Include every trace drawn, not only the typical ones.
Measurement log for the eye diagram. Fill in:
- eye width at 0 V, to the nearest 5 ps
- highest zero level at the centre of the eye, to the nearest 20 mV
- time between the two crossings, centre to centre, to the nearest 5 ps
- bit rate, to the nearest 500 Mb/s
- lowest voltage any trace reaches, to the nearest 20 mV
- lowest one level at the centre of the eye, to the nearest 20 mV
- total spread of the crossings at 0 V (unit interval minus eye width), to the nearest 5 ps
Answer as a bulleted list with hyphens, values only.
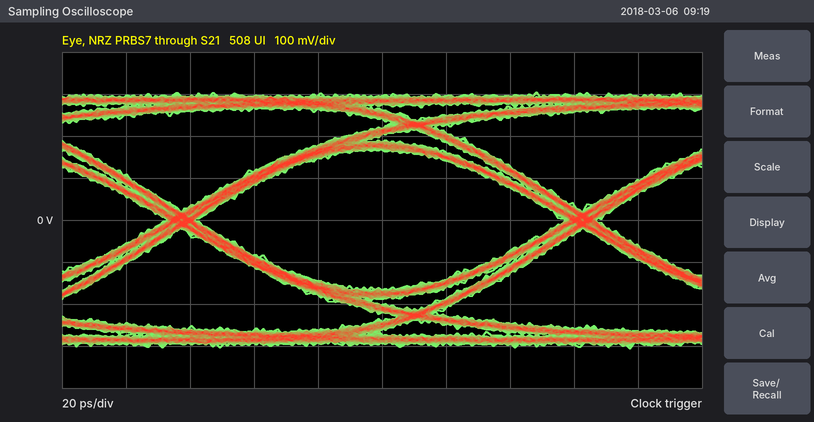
- 115 ps
- -160 mV
- 125 ps
- 8.0 Gb/s
- -300 mV
- 160 mV
- 10 ps
